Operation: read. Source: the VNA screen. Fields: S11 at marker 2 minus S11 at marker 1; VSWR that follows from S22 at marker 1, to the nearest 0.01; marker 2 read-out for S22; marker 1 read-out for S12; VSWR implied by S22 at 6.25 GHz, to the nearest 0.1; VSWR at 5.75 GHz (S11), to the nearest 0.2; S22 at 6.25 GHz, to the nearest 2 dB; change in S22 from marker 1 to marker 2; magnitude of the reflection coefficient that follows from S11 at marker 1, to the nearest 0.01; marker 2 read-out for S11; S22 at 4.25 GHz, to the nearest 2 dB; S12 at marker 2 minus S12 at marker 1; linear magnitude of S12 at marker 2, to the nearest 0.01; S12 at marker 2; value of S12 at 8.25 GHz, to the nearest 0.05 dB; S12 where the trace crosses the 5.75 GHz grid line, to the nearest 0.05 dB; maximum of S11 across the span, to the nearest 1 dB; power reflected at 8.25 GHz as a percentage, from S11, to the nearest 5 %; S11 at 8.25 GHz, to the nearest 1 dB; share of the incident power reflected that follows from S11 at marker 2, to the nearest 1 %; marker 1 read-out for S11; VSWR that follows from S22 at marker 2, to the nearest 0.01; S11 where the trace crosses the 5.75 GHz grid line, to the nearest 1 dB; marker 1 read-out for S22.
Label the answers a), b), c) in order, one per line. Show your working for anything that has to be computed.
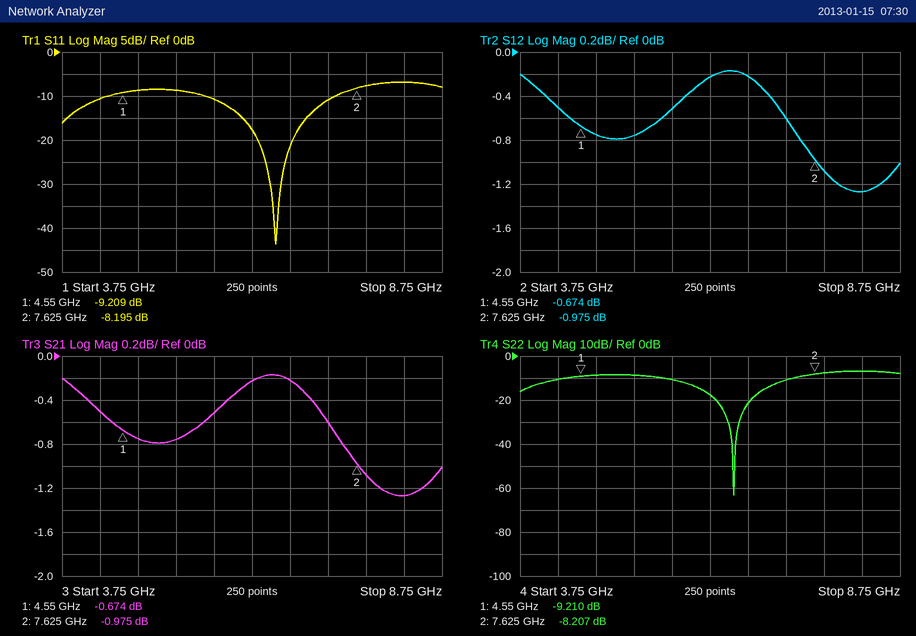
a) -8.195 − (-9.209) = 1.014 dB
b) (1 + 0.3463)/(1 − 0.3463) ≈ 2.06
c) -8.207 dB
d) -0.674 dB
e) |Γ| = 10^(-18/20) = 0.1259; VSWR = (1 + 0.1259)/(1 − 0.1259) ≈ 1.3
f) |Γ| = 10^(-11/20) = 0.2818; VSWR = (1 + 0.2818)/(1 − 0.2818) ≈ 1.8
g) -18 dB
h) -8.207 − (-9.21) = 1.003 dB
i) 10^(-9.209/20) ≈ 0.35
j) -8.195 dB
k) -10 dB
l) -0.975 − (-0.674) = -0.301 dB
m) 10^(-0.975/20) ≈ 0.89
n) -0.975 dB
o) -1.25 dB
p) -0.50 dB
q) -7 dB
r) 10^(-7/10) ≈ 20 %
s) -7 dB
t) 10^(-8.195/10) ≈ 15 %
u) -9.209 dB
v) (1 + 0.3887)/(1 − 0.3887) ≈ 2.27
w) -11 dB
x) -9.210 dB
